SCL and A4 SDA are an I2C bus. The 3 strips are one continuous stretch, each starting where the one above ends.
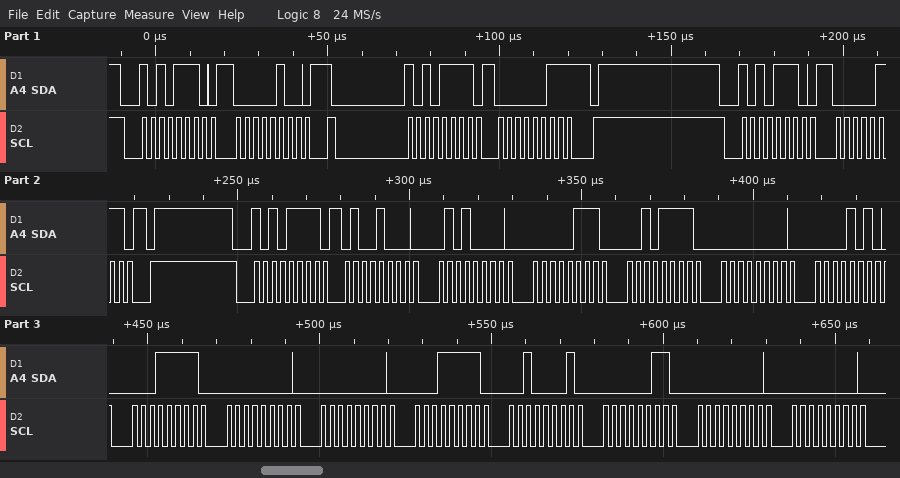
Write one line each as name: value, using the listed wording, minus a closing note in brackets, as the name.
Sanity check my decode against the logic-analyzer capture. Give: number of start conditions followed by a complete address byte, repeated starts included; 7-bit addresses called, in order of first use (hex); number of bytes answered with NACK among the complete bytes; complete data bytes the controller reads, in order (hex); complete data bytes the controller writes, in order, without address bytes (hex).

number of start conditions followed by a complete address byte, repeated starts included: 4
7-bit addresses called, in order of first use: 0x57
number of bytes answered with NACK among the complete bytes: 1
complete data bytes the controller reads, in order: 03 48 50 07 2F 00 0A 1F 00 00 1F 21 03 00 00
complete data bytes the controller writes, in order, without address bytes: 04 07
